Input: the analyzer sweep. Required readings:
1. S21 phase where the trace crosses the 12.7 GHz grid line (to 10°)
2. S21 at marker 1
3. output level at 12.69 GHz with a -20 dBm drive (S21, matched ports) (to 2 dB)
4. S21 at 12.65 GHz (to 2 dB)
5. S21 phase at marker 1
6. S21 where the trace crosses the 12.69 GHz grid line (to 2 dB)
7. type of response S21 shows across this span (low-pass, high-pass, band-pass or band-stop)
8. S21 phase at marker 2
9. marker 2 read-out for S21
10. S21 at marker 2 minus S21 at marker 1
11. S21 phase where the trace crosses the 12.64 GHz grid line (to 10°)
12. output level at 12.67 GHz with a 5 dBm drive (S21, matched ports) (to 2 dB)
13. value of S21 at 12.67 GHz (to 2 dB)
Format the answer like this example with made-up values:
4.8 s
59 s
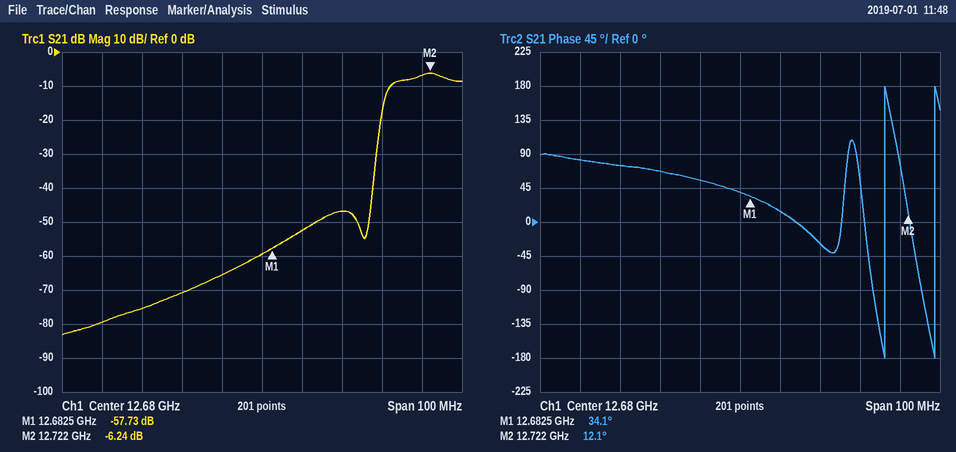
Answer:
-30°
-57.73 dB
-72 dBm
-76 dB
34.1°
-52 dB
high-pass
12.1°
-6.24 dB
51.49 dB
80°
-60 dBm
-66 dB
